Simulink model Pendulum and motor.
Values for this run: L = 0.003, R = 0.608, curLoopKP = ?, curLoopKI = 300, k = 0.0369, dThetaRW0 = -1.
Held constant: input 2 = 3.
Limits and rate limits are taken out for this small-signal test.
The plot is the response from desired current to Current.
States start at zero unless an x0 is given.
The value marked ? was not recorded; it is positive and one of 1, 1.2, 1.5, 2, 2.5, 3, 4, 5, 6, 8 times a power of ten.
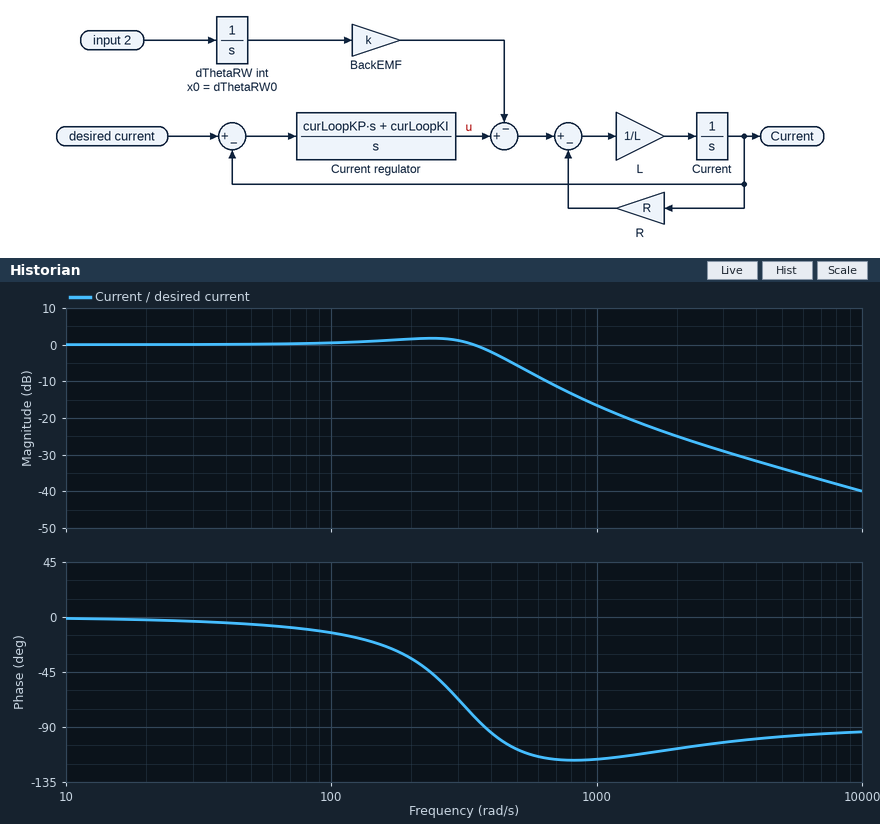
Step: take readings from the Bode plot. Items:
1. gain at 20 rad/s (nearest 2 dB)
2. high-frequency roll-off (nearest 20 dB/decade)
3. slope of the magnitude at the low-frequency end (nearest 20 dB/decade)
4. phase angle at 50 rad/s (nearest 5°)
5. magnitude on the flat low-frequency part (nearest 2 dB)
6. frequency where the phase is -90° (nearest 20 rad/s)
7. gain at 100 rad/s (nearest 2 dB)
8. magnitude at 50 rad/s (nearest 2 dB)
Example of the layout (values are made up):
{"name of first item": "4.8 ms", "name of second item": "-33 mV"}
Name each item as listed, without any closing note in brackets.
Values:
{"gain at 20 rad/s": "0 dB", "high-frequency roll-off": "-20 dB/decade", "slope of the magnitude at the low-frequency end": "0 dB/decade", "phase angle at 50 rad/s": "-5°", "magnitude on the flat low-frequency part": "0 dB", "frequency where the phase is -90°": "380 rad/s", "gain at 100 rad/s": "0 dB", "magnitude at 50 rad/s": "0 dB"}
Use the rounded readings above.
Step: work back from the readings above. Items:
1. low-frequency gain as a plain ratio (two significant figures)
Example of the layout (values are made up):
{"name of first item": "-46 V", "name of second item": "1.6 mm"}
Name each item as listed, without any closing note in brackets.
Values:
{"low-frequency gain as a plain ratio": "1.0"}
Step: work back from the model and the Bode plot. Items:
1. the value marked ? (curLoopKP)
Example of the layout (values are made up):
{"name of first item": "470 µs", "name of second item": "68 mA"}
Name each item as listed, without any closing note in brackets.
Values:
{"the value marked ?": "0.3"}
